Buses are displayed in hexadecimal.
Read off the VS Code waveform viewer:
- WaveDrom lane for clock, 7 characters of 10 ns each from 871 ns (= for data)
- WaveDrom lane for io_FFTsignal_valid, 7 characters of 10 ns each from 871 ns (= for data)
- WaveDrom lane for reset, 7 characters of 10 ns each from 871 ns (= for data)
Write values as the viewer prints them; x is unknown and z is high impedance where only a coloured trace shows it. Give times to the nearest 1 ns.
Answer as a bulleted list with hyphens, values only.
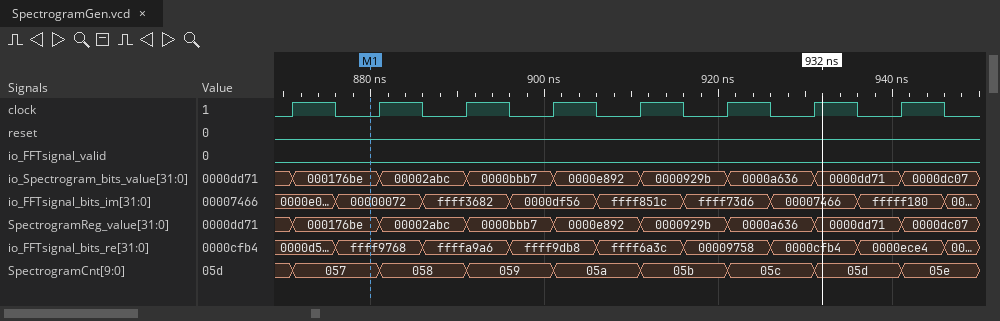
- {name: 'clock', wave: 'p......'}
- {name: 'io_FFTsignal_valid', wave: '0......'}
- {name: 'reset', wave: '0......'}
